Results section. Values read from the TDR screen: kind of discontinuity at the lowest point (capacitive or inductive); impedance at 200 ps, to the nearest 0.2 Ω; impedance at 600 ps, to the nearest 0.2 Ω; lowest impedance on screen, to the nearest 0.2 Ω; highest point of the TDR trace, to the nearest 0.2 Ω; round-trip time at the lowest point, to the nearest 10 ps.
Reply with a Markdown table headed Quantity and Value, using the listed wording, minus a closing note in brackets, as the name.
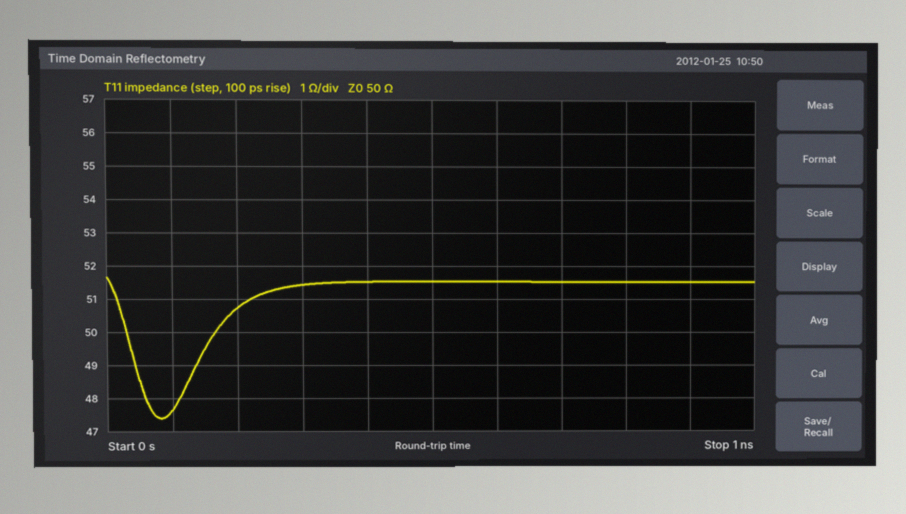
| Quantity | Value |
|---|---|
| kind of discontinuity at the lowest point | capacitive |
| impedance at 200 ps, to the nearest 0.2 Ω | 50.8 Ω |
| impedance at 600 ps, to the nearest 0.2 Ω | 51.6 Ω |
| lowest impedance on screen, to the nearest 0.2 Ω | 47.4 Ω |
| highest point of the TDR trace, to the nearest 0.2 Ω | 51.6 Ω |
| round-trip time at the lowest point, to the nearest 10 ps | 80 ps |
